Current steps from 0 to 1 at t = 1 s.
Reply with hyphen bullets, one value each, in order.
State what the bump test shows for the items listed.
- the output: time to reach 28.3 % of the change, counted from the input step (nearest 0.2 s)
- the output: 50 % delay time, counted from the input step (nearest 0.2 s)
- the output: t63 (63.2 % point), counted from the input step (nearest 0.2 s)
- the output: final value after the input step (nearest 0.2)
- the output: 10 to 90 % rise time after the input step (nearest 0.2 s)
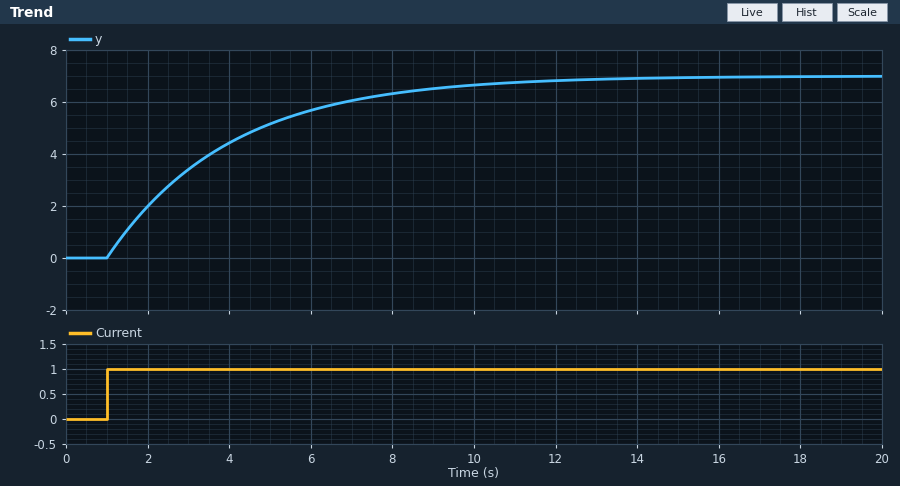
- 1.0 s
- 2.0 s
- 3.0 s
- 7.0
- 6.6 s
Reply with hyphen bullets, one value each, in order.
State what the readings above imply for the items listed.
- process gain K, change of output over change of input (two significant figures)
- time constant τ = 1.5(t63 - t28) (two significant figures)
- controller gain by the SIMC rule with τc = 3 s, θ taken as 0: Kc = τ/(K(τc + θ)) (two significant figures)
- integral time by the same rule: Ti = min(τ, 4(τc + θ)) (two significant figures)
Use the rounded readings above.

- 7.0
- 3.0 s
- 0.14
- 3.0 s
